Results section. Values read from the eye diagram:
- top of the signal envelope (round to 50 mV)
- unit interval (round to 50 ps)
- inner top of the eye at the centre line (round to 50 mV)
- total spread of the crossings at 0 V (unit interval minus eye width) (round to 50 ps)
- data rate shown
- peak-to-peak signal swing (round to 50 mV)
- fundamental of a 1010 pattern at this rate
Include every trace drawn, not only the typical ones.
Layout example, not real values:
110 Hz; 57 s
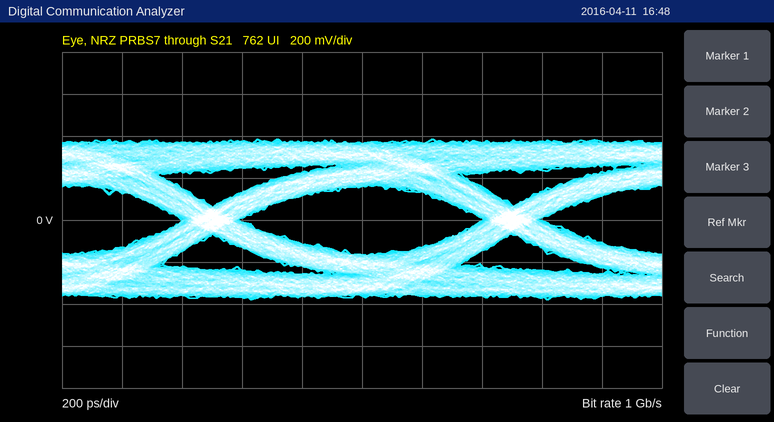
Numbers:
400 mV; 1.00 ns; 150 mV; 200 ps; 1 Gb/s; 750 mV; 500 MHz
